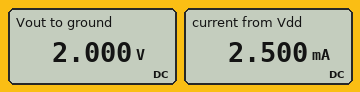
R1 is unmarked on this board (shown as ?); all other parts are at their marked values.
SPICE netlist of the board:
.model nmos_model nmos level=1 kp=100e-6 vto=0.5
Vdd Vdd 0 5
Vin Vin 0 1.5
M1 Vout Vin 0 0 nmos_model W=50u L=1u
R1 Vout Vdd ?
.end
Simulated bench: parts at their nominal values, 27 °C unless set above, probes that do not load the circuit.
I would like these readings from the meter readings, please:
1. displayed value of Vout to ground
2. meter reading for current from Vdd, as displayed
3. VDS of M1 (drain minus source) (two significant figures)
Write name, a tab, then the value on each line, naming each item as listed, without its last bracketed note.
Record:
displayed value of Vout to ground	2.000 V
meter reading for current from Vdd, as displayed	2.500 mA
VDS of M1 (drain minus source)	2.0 V
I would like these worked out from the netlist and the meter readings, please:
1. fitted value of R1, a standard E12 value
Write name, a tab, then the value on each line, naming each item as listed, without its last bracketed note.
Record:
fitted value of R1, a standard E12 value	1.2 kΩ
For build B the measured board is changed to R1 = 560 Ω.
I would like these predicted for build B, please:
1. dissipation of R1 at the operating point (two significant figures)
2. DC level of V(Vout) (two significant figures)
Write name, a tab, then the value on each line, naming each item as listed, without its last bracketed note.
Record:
dissipation of R1 at the operating point	3.5 mW
DC level of V(Vout)	3.6 V
